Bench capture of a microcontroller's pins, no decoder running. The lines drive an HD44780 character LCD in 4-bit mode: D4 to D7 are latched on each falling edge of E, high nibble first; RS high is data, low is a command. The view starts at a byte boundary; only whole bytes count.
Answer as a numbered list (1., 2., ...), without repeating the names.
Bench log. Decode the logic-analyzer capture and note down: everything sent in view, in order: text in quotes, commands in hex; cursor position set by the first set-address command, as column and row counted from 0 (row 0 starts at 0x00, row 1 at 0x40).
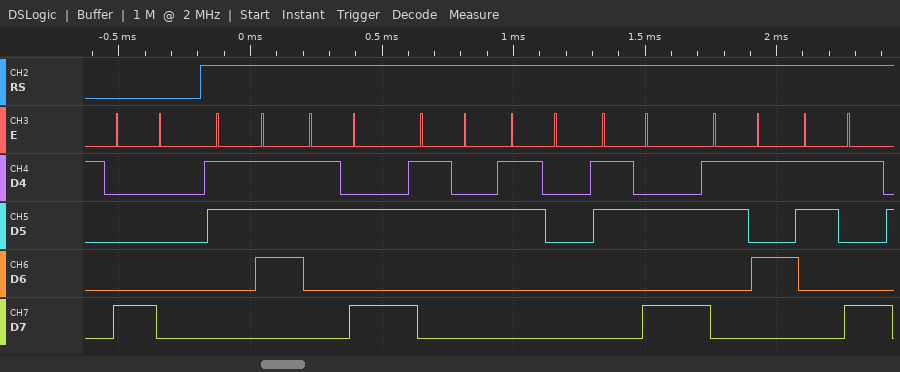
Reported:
1. 0x80 "7:20:59"
2. column 0, row 0
